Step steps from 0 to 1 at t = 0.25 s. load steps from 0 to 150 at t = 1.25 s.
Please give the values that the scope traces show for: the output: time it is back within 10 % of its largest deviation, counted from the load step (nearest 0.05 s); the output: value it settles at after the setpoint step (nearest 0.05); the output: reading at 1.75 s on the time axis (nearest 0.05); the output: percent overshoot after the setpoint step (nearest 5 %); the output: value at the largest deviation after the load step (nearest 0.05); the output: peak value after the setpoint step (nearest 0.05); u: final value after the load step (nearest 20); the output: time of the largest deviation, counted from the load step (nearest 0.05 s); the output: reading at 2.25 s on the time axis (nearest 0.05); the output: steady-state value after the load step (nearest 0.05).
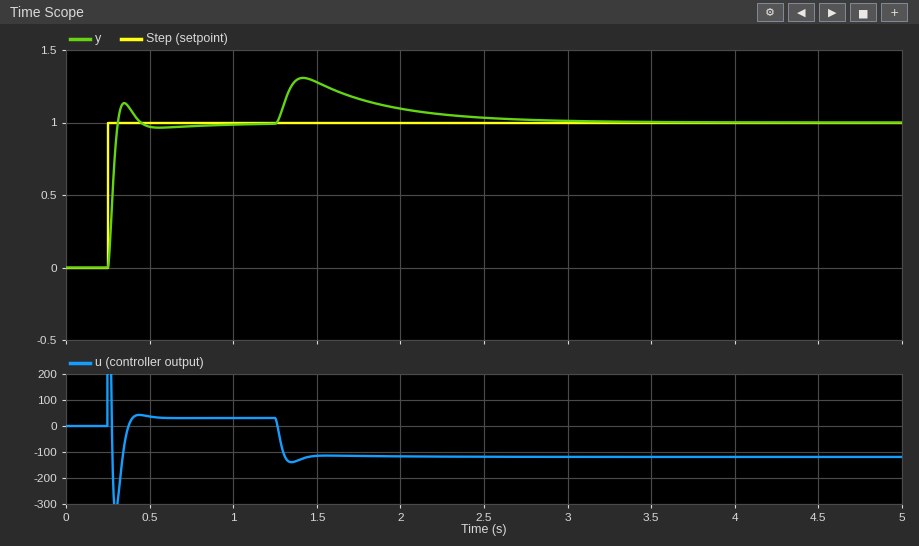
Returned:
1.25 s
1.00
1.15
15 %
1.30
1.15
-120
0.15 s
1.05
1.00
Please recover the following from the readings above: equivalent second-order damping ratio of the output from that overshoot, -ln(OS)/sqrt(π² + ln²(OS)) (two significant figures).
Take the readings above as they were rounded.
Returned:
0.52
